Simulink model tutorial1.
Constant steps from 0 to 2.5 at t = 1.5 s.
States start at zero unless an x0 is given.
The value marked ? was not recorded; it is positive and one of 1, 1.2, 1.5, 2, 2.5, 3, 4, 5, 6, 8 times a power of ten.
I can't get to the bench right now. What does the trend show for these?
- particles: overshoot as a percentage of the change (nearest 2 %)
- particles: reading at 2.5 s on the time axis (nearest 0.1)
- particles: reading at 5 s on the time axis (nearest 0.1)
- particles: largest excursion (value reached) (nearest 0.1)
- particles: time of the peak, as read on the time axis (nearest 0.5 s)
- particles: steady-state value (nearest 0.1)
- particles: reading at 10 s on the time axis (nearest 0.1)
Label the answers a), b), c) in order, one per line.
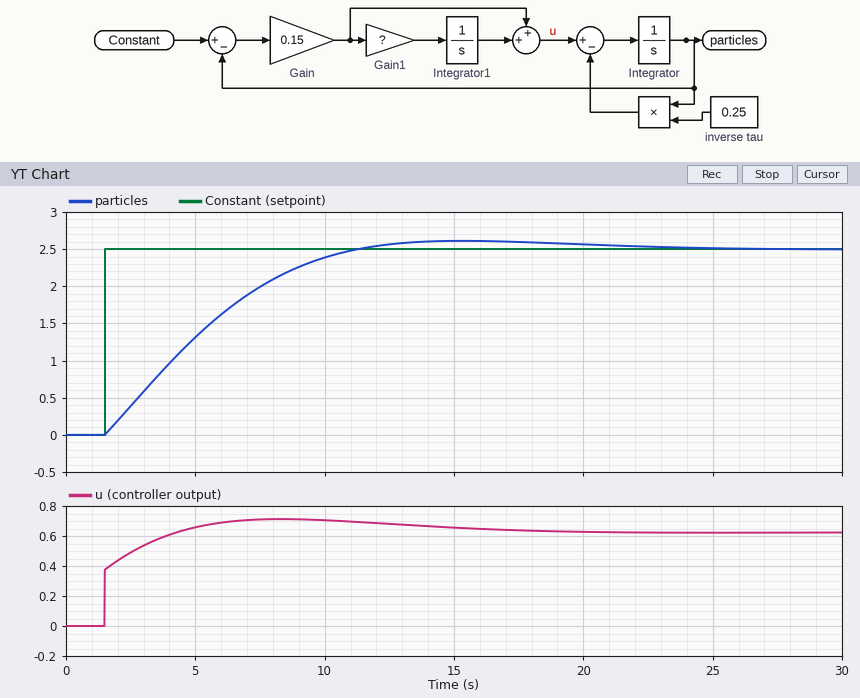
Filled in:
a) 4 %
b) 0.4
c) 1.3
d) 2.6
e) 15.5 s
f) 2.5
g) 2.4
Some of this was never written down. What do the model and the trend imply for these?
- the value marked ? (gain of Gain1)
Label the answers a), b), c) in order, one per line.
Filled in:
a) 0.5
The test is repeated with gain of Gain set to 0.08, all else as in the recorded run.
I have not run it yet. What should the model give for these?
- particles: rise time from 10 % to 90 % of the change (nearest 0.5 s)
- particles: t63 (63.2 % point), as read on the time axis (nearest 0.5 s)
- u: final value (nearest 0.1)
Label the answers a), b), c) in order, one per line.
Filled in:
a) 12.0 s
b) 9.0 s
c) 0.6
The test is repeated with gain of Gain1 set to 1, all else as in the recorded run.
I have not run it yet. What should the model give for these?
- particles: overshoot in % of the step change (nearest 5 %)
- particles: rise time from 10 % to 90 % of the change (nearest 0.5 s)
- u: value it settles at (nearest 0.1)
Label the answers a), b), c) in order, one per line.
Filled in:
a) 15 %
b) 4.0 s
c) 0.6
